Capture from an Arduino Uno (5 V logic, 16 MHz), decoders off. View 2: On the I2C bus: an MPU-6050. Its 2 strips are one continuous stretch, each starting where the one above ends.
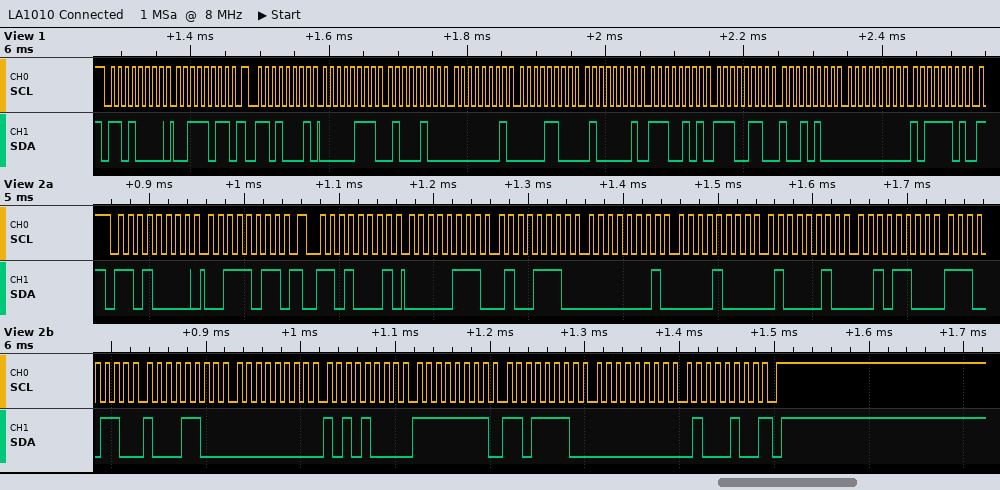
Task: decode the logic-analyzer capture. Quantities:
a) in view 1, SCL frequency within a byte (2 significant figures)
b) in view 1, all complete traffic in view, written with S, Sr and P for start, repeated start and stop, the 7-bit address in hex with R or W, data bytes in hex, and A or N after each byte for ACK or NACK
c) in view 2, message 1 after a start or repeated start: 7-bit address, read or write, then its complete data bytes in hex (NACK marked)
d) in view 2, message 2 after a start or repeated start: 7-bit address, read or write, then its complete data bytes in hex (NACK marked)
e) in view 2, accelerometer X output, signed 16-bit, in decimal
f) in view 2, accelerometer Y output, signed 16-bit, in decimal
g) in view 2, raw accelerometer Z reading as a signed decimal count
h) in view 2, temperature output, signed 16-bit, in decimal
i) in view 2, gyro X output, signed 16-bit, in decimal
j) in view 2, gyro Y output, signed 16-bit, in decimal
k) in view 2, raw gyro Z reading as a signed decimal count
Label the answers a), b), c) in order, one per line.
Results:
a) 100 kHz
b) S 68W A 3B A Sr 68R A 07 A 44 A 01 A 0C A 41 A E5 A E6 A 94 A 00 A BD A
c) 0x68 write: 3B
d) 0x68 read: 07 4E 01 08 42 2C E6 8C 00 A8 FF DE 00 44 NACK
e) 1870
f) 264
g) 16940
h) -6516
i) 168
j) -34
k) 68
